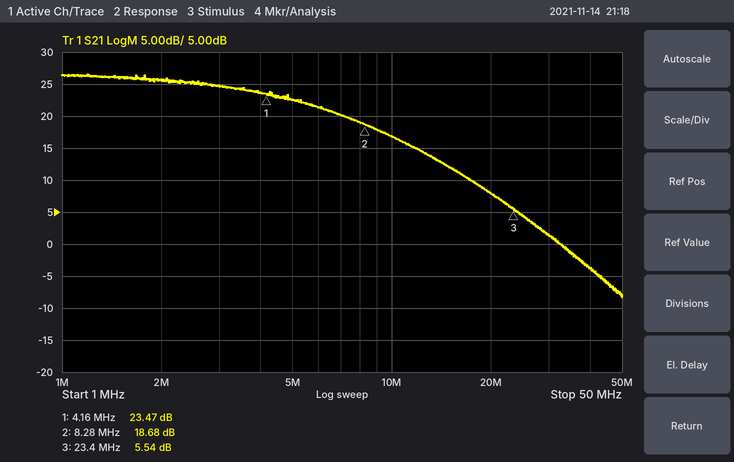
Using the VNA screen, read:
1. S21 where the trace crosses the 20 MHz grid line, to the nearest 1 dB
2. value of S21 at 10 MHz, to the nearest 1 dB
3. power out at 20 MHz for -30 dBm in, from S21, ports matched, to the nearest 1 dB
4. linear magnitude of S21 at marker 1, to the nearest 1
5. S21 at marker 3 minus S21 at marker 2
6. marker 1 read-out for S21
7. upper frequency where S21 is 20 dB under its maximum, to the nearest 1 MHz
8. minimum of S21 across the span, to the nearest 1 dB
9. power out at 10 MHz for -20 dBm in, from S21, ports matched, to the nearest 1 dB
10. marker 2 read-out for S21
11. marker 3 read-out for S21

8 dB
17 dB
-22 dBm
15
-13.14 dB
23.47 dB
22 MHz
-8 dB
-3 dBm
18.68 dB
5.54 dB
